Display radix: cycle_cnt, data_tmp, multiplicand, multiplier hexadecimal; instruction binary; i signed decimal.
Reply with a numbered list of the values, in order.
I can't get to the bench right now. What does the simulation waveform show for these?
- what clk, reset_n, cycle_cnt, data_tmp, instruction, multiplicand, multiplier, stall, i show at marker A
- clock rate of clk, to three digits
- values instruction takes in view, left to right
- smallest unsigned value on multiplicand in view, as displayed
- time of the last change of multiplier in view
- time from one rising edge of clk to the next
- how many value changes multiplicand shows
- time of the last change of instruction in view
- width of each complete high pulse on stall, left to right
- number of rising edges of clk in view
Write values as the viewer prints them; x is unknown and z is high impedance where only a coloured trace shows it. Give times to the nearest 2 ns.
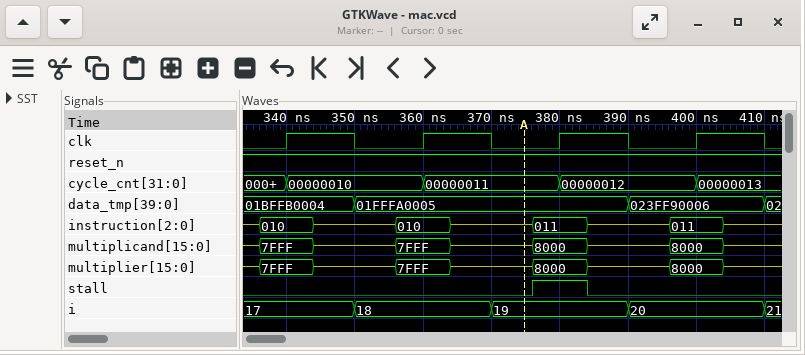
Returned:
1. clk=0, reset_n=1, cycle_cnt=00000011, data_tmp=01FFFA0005, instruction=z, multiplicand=z, multiplier=z, stall=0, i=19
2. 50.0 MHz
3. z, 010, z, 010, z, 011, z, 011, z
4. 7FFF
5. 404 ns
6. 20 ns
7. 8
8. 404 ns
9. 8 ns
10. 4
